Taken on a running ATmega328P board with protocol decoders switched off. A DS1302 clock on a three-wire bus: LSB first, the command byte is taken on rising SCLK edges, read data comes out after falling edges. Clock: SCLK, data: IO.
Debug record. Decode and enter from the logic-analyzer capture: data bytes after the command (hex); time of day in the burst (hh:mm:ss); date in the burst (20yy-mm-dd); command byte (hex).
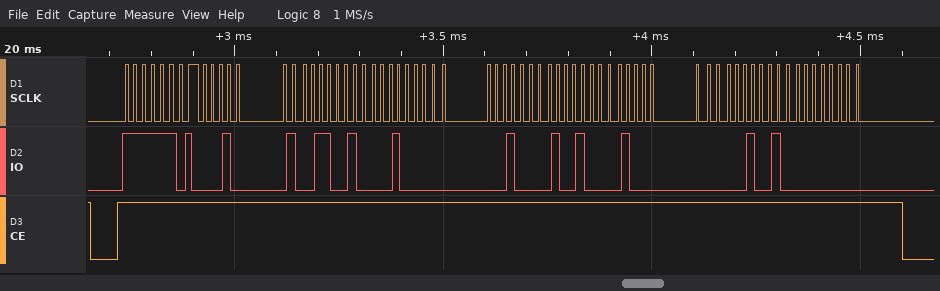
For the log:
48 26 04 08 09 01 24 00
04:26:48
2024-09-08
0xBF
